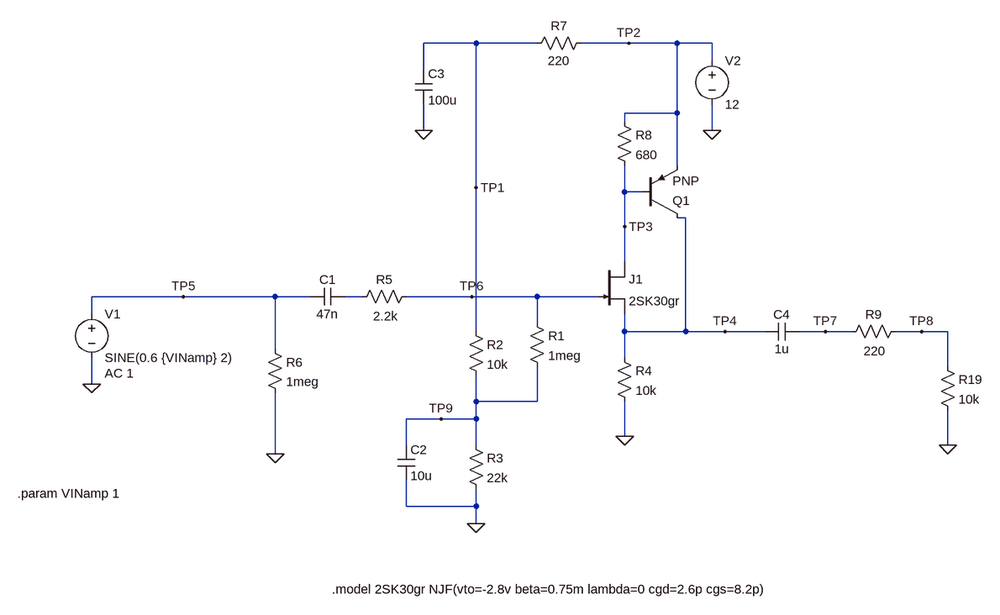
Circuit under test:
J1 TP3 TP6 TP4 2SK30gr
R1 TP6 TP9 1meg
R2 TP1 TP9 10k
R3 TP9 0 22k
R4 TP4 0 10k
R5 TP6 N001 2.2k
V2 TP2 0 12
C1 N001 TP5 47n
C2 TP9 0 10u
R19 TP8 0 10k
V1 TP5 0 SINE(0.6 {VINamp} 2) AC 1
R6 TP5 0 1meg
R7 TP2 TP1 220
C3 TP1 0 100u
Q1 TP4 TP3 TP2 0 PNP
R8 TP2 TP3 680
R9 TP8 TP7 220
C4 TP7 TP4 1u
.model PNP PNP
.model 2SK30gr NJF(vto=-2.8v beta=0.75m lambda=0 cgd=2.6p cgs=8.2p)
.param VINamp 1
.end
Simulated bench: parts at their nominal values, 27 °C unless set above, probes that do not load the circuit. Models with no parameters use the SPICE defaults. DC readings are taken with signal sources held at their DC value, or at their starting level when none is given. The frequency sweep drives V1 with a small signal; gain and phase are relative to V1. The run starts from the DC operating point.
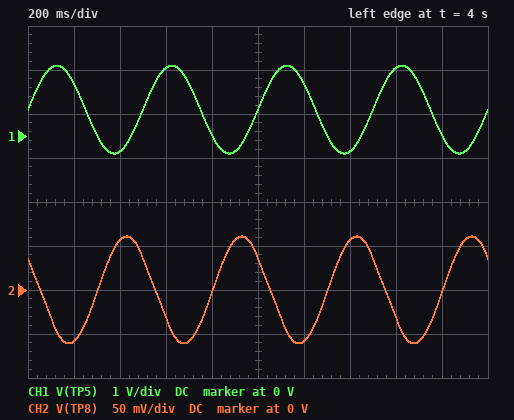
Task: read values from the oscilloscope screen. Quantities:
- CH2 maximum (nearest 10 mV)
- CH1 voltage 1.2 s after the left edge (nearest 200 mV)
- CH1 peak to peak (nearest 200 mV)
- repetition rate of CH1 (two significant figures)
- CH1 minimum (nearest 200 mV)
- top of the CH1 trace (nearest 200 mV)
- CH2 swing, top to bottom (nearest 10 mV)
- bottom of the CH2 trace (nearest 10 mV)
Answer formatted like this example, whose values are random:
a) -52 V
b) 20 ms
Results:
a) 60 mV
b) 1.2 V
c) 2.0 V
d) 2.0 Hz
e) -400 mV
f) 1.6 V
g) 120 mV
h) -60 mV
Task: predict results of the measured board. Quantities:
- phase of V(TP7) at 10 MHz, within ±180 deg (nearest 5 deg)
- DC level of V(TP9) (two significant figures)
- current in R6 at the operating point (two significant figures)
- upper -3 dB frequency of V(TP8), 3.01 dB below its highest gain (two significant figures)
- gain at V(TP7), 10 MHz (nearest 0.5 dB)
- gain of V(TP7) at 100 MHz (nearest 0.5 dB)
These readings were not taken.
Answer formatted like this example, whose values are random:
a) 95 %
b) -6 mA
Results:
a) -15 deg
b) 8.2 V
c) 600 nA
d) 34 MHz
e) -1.0 dB
f) -10.5 dB
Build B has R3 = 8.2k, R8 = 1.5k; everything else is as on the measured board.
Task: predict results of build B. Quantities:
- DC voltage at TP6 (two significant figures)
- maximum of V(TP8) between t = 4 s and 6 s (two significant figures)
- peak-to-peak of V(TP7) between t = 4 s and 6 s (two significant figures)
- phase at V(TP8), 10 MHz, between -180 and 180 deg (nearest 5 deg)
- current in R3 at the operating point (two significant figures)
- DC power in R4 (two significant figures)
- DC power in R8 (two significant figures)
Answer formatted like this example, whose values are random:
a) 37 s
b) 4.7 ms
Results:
a) 5.3 V
b) 63 mV
c) 130 mV
d) -10 deg
e) 650 µA
f) 5.4 mW
g) 360 µW
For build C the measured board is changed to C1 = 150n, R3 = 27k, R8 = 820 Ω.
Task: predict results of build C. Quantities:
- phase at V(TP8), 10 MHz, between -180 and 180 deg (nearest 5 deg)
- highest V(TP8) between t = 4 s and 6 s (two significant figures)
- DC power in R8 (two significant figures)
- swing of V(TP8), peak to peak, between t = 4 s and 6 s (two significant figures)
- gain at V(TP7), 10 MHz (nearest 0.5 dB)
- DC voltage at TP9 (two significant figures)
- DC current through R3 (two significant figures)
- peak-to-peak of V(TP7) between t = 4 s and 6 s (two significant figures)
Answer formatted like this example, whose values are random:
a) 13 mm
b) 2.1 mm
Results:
a) -20 deg
b) 100 mV
c) 640 µW
d) 200 mV
e) -2.5 dB
f) 8.7 V
g) 320 µA
h) 210 mV
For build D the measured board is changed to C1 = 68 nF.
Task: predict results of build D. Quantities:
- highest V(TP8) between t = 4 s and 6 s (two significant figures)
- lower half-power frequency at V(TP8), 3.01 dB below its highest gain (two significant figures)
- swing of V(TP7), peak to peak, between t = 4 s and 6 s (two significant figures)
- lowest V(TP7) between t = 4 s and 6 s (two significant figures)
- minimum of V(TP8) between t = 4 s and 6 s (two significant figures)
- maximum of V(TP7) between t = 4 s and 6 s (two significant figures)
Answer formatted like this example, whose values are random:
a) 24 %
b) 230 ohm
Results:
a) 78 mV
b) 15 Hz
c) 160 mV
d) -79 mV
e) -77 mV
f) 79 mV
